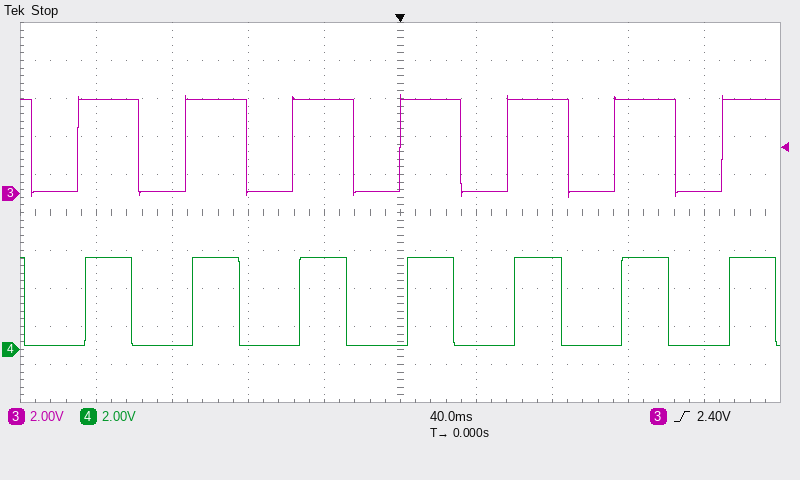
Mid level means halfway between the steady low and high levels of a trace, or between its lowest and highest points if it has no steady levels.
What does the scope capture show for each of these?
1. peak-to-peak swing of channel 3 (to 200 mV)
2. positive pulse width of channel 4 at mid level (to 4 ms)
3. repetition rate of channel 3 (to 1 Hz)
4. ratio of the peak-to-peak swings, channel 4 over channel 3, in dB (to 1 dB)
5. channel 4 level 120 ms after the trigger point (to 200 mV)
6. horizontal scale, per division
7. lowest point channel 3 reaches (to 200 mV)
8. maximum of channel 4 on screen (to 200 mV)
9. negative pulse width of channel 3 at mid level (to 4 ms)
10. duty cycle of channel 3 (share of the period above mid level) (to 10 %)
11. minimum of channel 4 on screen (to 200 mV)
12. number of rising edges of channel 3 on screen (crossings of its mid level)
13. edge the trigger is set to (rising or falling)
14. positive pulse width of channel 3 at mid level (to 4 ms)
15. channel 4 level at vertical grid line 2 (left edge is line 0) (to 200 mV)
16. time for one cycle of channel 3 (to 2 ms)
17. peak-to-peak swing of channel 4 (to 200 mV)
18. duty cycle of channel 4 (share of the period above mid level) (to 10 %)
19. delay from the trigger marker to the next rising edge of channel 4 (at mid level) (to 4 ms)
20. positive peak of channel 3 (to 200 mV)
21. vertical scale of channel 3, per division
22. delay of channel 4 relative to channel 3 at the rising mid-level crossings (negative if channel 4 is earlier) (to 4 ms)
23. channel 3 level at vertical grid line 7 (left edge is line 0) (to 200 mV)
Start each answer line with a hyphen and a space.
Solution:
- 5.4 V
- 24 ms
- 18 Hz
- -1 dB
- 4.8 V
- 40 ms
- -200 mV
- 4.8 V
- 24 ms
- 60 %
- 200 mV
- 7
- rising
- 32 ms
- 200 mV
- 56 ms
- 4.6 V
- 40 %
- 4 ms
- 5.2 V
- 2 V
- +4 ms
- 5.0 V
